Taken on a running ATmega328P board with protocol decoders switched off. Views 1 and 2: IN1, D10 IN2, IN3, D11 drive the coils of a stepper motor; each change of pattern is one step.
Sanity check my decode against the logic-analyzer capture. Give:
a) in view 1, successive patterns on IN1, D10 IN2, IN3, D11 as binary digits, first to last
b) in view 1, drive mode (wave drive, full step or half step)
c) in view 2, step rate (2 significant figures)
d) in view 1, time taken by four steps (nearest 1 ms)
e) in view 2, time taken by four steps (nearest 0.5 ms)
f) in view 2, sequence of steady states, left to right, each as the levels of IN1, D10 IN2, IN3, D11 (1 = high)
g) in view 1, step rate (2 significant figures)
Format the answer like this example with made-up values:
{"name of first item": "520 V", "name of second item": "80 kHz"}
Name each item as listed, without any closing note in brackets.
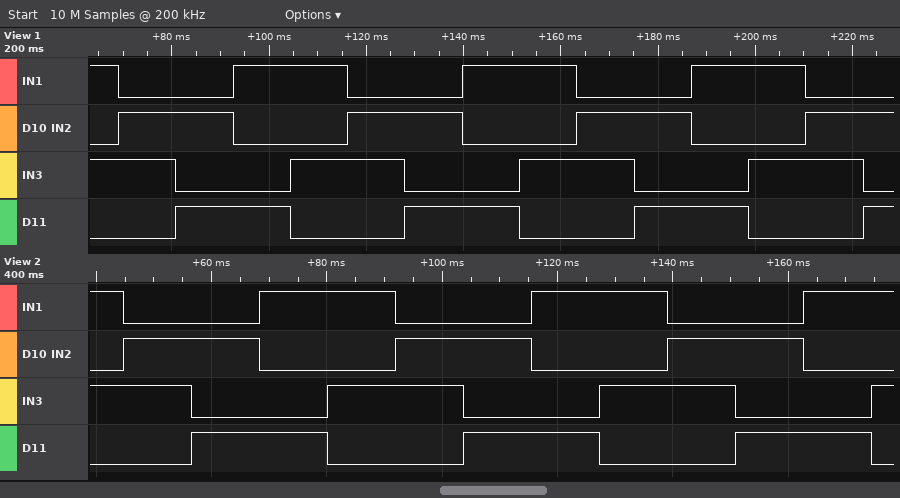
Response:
{"in view 1, successive patterns on IN1, D10 IN2, IN3, D11 as binary digits, first to last": "1010 0110 0101 1001 1010 0110 0101 1001 1010 0110 0101 1001 1010 0110 0101", "in view 1, drive mode": "full step", "in view 2, step rate": "85 steps/s", "in view 1, time taken by four steps": "47 ms", "in view 2, time taken by four steps": "47.0 ms", "in view 2, sequence of steady states, left to right, each as the levels of IN1, D10 IN2, IN3, D11": "1010 0110 0101 1001 1010 0110 0101 1001 1010 0110 0101 1001 1010", "in view 1, step rate": "85 steps/s"}
